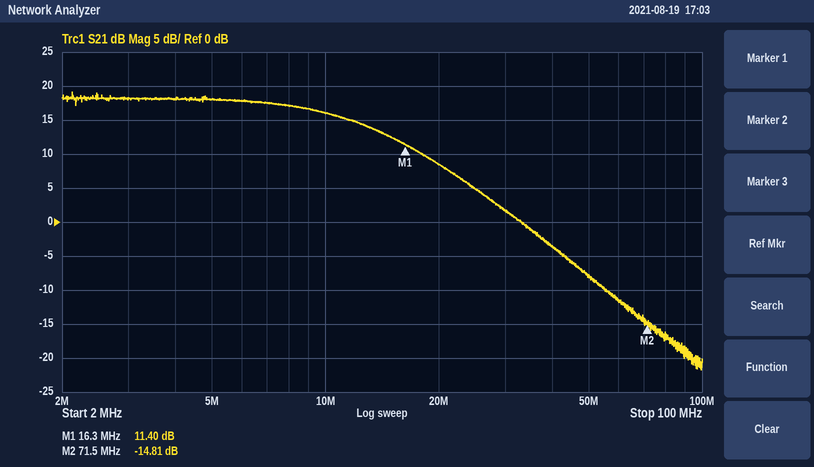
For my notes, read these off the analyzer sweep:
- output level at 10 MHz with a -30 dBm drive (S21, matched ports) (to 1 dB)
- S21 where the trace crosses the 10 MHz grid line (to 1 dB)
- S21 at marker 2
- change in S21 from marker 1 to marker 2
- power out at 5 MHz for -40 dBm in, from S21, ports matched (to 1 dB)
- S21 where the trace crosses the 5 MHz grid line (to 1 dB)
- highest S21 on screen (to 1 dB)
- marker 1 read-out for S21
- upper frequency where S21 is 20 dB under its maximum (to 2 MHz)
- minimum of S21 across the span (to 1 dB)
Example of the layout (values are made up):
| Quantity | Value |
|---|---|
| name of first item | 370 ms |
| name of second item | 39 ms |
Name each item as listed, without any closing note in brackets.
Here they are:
| Quantity | Value |
|---|---|
| output level at 10 MHz with a -30 dBm drive (S21, matched ports) | -14 dBm |
| S21 where the trace crosses the 10 MHz grid line | 16 dB |
| S21 at marker 2 | -14.81 dB |
| change in S21 from marker 1 to marker 2 | -26.21 dB |
| power out at 5 MHz for -40 dBm in, from S21, ports matched | -22 dBm |
| S21 where the trace crosses the 5 MHz grid line | 18 dB |
| highest S21 on screen | 19 dB |
| marker 1 read-out for S21 | 11.40 dB |
| upper frequency where S21 is 20 dB under its maximum | 34 MHz |
| minimum of S21 across the span | -22 dB |
